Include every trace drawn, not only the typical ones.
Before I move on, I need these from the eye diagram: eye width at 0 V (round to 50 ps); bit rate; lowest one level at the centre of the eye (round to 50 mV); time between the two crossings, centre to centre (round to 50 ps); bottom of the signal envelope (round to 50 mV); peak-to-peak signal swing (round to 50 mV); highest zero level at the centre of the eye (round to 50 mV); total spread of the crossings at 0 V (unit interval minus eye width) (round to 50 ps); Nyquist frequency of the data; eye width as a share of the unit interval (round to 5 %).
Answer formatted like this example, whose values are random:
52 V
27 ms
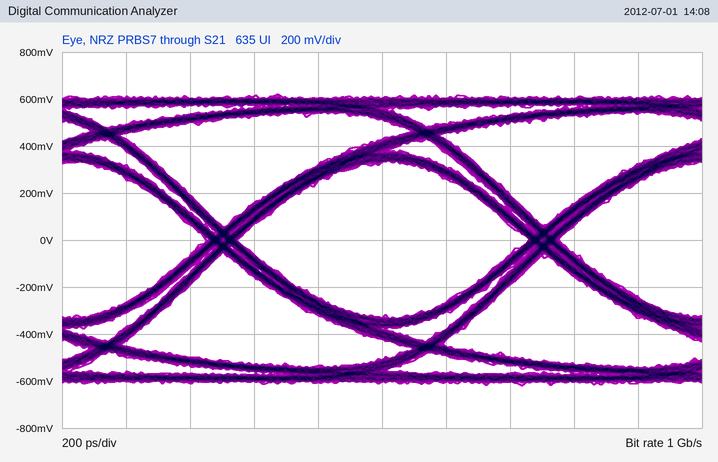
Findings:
900 ps
1 Gb/s
350 mV
1.00 ns
-600 mV
1.25 V
-350 mV
100 ps
500 MHz
90 %
